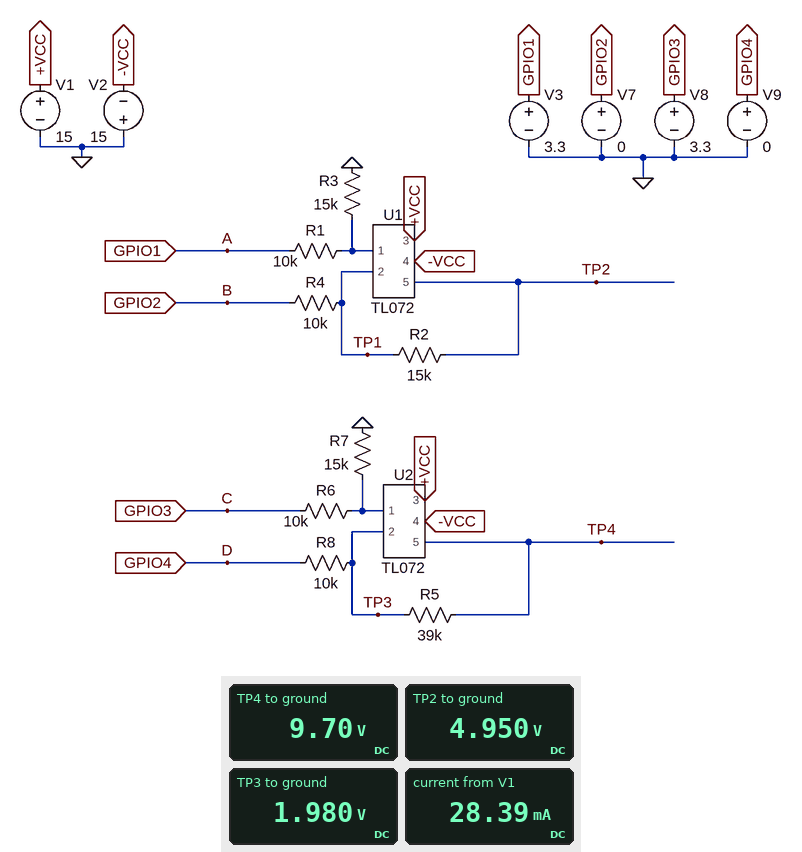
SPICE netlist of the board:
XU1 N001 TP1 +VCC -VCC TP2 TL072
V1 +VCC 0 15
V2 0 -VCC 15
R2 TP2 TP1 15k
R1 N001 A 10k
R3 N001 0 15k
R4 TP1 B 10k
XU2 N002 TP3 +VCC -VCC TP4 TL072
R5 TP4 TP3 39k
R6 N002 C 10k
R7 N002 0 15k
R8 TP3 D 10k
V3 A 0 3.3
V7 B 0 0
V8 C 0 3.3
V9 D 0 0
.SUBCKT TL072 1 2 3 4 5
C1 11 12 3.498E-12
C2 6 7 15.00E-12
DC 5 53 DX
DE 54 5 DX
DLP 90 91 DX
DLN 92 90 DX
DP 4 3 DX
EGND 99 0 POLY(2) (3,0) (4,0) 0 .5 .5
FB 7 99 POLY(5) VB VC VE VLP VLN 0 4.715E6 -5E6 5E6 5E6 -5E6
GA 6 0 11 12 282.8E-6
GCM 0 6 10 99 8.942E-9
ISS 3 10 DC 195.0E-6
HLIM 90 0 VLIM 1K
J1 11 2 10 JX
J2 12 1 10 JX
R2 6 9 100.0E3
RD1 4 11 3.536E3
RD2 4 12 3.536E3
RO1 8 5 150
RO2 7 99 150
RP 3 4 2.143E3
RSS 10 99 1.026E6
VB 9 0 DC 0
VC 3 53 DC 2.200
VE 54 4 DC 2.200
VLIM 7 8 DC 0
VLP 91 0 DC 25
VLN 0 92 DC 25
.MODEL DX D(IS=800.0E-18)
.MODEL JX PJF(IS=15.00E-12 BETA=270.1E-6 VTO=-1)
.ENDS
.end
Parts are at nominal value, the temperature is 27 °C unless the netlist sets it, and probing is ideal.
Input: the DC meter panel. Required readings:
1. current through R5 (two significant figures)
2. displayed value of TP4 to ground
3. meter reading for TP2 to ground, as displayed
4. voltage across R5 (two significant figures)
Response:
200 µA
9.70 V
4.950 V
7.7 V
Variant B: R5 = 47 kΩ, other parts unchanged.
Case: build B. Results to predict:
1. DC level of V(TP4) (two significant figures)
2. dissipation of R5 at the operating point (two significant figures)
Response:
11 V
1.8 mW
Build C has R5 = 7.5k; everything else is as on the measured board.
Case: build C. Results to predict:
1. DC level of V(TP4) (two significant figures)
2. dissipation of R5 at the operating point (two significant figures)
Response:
3.5 V
290 µW
